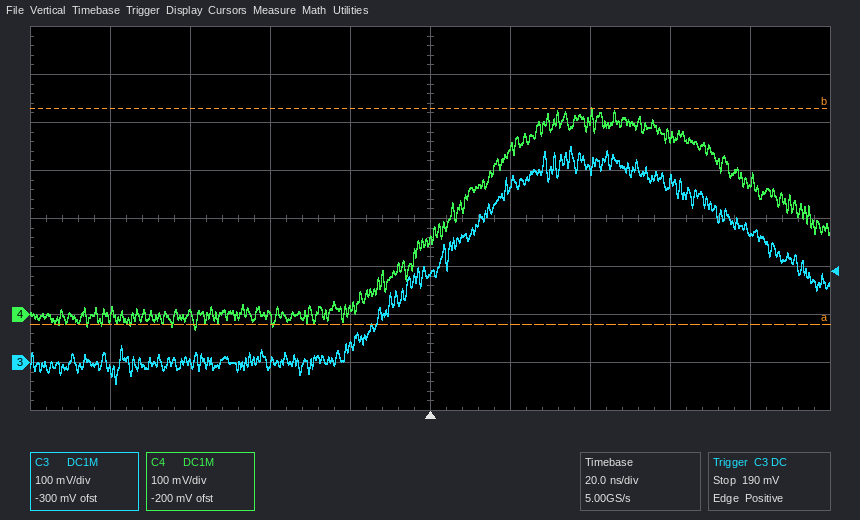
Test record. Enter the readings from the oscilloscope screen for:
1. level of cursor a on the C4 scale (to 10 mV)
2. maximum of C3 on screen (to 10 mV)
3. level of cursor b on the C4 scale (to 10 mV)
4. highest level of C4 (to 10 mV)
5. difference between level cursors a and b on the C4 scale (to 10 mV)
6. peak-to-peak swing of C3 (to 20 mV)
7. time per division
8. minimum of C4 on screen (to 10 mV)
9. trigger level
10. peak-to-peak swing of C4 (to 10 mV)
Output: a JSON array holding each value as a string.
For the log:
["-20 mV", "450 mV", "430 mV", "430 mV", "450 mV", "500 mV", "20 ns", "-30 mV", "190 mV", "460 mV"]
